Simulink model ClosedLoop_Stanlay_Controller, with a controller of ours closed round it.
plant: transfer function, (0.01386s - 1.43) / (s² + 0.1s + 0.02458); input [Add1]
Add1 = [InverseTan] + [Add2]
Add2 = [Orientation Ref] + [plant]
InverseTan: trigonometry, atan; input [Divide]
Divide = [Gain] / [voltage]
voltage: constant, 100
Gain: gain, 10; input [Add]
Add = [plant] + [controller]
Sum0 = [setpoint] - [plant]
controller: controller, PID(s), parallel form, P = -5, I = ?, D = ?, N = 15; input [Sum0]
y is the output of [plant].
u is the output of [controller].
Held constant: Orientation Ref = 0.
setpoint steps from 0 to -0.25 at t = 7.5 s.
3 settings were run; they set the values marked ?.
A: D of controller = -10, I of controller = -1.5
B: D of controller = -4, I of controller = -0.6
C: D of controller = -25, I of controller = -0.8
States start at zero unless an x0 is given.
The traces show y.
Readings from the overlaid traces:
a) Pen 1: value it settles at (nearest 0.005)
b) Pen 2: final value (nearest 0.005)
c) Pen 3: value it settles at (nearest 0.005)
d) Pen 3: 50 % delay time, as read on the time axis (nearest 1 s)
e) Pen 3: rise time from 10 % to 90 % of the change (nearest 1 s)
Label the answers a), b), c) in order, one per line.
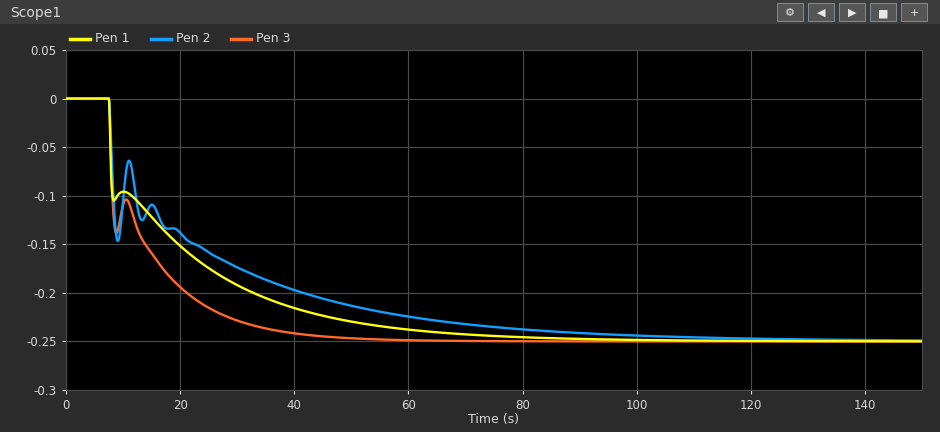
a) -0.250
b) -0.250
c) -0.250
d) 8 s
e) 21 s
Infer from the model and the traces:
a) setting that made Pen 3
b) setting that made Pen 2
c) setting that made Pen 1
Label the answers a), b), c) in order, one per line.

a) A
b) B
c) C
